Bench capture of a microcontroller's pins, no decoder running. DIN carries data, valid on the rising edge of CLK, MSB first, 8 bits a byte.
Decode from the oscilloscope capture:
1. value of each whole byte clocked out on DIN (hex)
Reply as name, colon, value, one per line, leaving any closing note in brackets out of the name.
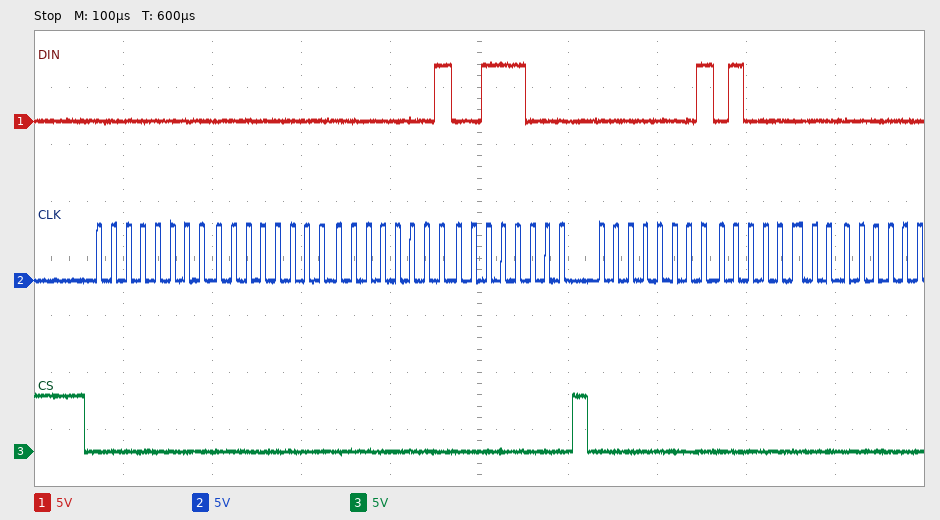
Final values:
value of each whole byte clocked out on DIN: 00 00 01 38 01 40
